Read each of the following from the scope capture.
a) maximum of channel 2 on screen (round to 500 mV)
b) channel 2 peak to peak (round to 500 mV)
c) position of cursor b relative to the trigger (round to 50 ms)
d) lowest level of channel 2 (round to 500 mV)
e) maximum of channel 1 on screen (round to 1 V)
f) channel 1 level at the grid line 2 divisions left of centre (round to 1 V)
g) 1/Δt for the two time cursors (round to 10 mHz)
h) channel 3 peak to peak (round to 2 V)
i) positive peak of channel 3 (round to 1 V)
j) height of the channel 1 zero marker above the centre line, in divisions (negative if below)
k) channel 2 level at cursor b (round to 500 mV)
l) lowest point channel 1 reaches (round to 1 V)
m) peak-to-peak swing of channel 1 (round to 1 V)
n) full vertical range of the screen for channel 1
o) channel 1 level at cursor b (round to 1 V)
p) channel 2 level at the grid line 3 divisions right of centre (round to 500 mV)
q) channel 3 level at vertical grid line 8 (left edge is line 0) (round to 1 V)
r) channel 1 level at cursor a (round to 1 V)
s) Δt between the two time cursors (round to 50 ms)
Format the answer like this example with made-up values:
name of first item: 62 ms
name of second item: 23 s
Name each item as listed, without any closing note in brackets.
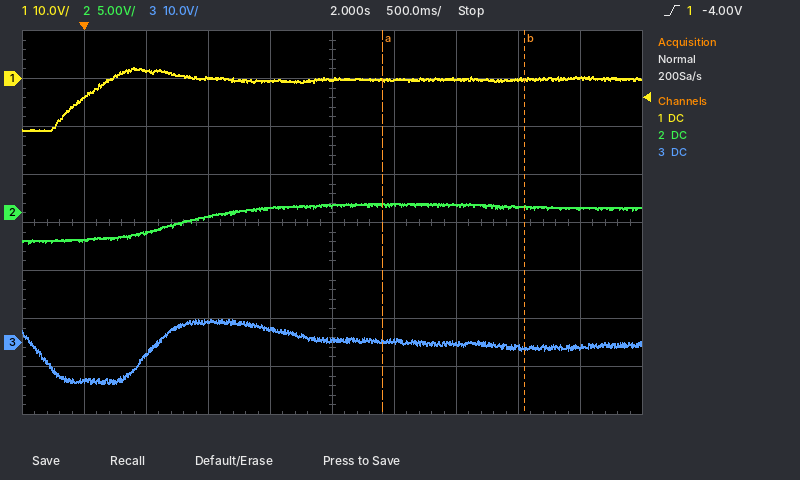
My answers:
maximum of channel 2 on screen: 1.0 V
channel 2 peak to peak: 4.0 V
position of cursor b relative to the trigger: +3.55 s
lowest level of channel 2: -3.0 V
maximum of channel 1 on screen: 2 V
channel 1 level at the grid line 2 divisions left of centre: 0 V
1/Δt for the two time cursors: 870 mHz
channel 3 peak to peak: 14 V
positive peak of channel 3: 5 V
height of the channel 1 zero marker above the centre line, in divisions: +3.0 div
channel 2 level at cursor b: 500 mV
lowest point channel 1 reaches: -11 V
peak-to-peak swing of channel 1: 13 V
full vertical range of the screen for channel 1: 80 V
channel 1 level at cursor b: 0 V
channel 2 level at the grid line 3 divisions right of centre: 500 mV
channel 3 level at vertical grid line 8 (left edge is line 0): -1 V
channel 1 level at cursor a: 0 V
Δt between the two time cursors: 1.15 s
